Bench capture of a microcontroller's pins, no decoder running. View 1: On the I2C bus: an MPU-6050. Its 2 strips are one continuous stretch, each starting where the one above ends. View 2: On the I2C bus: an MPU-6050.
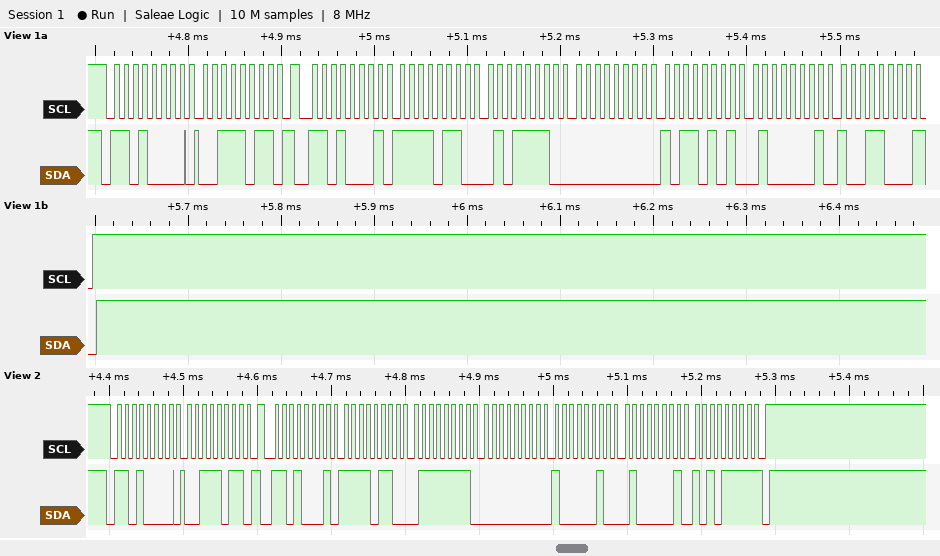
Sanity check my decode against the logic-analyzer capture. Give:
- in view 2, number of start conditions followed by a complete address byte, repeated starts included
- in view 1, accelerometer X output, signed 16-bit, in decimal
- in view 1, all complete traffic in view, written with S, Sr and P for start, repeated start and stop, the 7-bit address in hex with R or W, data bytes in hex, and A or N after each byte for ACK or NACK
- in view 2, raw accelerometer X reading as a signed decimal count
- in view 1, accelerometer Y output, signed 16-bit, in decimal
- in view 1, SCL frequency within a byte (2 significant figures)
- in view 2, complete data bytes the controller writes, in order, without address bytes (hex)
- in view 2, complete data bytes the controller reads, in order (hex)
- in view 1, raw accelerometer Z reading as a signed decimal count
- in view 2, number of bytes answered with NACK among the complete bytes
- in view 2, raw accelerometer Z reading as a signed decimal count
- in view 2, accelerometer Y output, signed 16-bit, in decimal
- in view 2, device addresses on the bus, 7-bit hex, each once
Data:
2
-2466
S 68W A 3B A Sr 68R A F6 A 5E A 00 A B5 A 41 A 98 N P
-2433
181
100 kHz
3B
F6 7F 00 82 41 AF
16792
1
16815
130
0x68
